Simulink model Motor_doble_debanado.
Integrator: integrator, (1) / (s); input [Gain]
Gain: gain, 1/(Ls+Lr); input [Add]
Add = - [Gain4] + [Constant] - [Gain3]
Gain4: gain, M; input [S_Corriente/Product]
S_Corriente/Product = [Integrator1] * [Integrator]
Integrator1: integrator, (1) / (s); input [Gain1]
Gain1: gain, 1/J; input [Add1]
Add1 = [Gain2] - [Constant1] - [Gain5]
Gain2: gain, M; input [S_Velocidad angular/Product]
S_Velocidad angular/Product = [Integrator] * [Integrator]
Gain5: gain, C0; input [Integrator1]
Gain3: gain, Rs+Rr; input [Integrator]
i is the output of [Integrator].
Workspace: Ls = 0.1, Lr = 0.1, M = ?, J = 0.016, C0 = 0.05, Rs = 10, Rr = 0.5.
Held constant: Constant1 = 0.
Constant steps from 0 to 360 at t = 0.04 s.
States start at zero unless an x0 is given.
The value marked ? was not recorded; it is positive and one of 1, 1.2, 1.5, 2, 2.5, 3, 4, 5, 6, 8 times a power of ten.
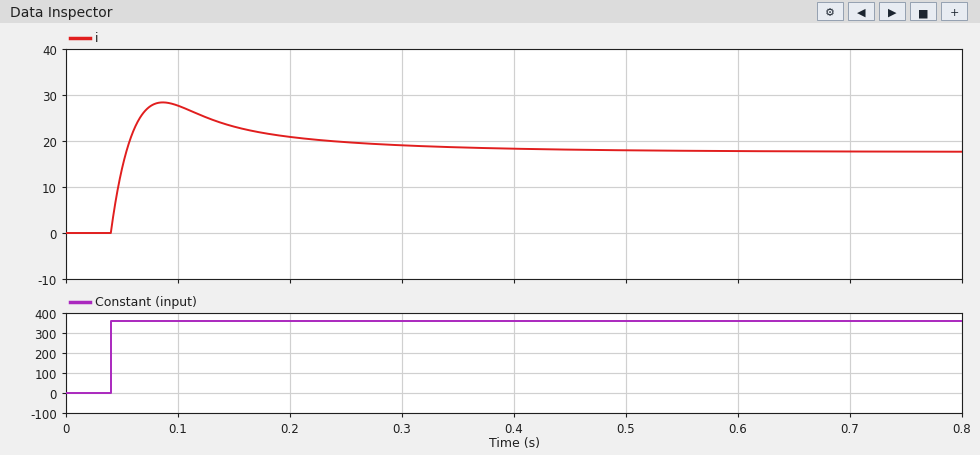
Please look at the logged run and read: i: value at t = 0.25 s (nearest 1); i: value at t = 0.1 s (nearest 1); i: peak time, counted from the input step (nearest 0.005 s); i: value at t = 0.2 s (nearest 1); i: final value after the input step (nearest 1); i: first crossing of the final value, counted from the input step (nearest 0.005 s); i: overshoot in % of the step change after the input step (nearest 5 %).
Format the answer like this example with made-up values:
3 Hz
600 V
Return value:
20
28
0.045 s
21
18
0.015 s
60 %
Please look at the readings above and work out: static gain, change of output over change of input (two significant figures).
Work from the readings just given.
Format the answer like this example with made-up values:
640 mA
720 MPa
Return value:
0.050
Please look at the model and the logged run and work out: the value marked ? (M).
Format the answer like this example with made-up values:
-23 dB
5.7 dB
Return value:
0.04
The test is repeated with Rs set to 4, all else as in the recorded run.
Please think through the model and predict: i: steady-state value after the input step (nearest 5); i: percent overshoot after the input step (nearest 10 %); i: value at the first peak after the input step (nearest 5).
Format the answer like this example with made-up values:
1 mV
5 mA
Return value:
20
110 %
40
